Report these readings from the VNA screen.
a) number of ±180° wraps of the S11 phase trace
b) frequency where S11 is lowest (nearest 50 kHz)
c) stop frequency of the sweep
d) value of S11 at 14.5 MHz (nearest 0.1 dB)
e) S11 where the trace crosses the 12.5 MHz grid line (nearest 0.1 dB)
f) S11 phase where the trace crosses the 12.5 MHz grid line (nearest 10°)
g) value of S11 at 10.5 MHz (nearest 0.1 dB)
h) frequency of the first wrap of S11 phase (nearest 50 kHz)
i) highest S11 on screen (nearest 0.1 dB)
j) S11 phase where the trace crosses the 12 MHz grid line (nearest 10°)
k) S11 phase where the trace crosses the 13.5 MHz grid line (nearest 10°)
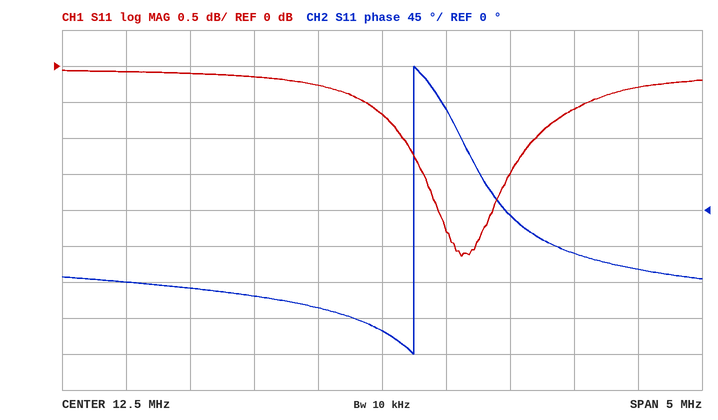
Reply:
1
13.10 MHz
15 MHz
-0.3 dB
-0.7 dB
-150°
-0.1 dB
12.75 MHz
-0.1 dB
-120°
-10°
